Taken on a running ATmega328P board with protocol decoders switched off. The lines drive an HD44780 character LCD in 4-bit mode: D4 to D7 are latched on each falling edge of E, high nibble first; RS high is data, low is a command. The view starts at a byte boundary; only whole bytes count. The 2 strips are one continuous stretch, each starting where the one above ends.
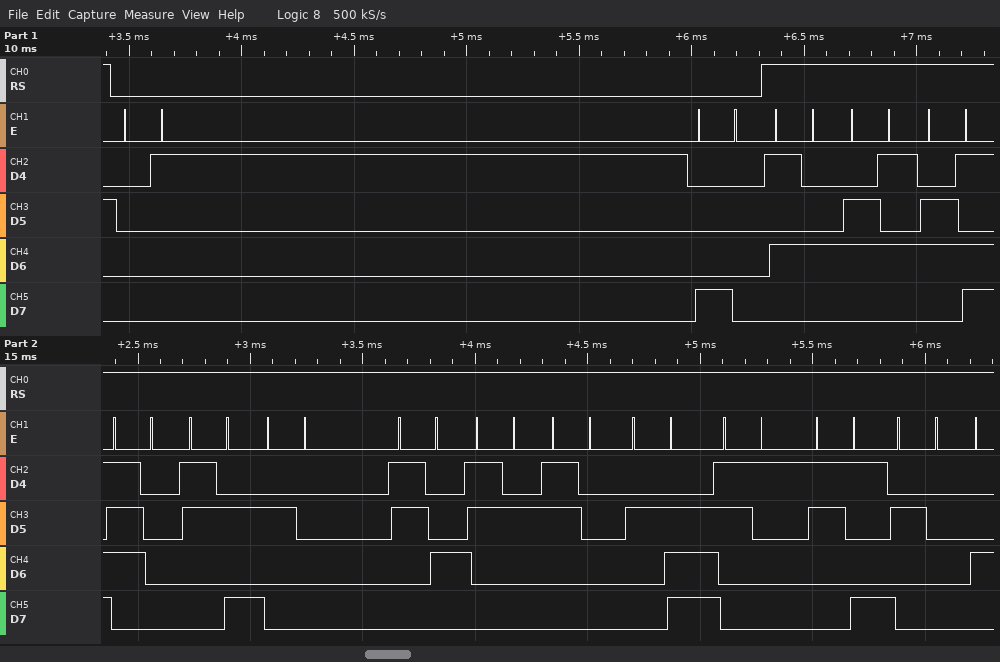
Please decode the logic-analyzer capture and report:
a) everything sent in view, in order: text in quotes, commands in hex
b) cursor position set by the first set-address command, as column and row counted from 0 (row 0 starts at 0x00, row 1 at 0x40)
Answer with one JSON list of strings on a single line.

["0x01 0x80 \"Temp: 420.19 \"", "column 0, row 0"]
